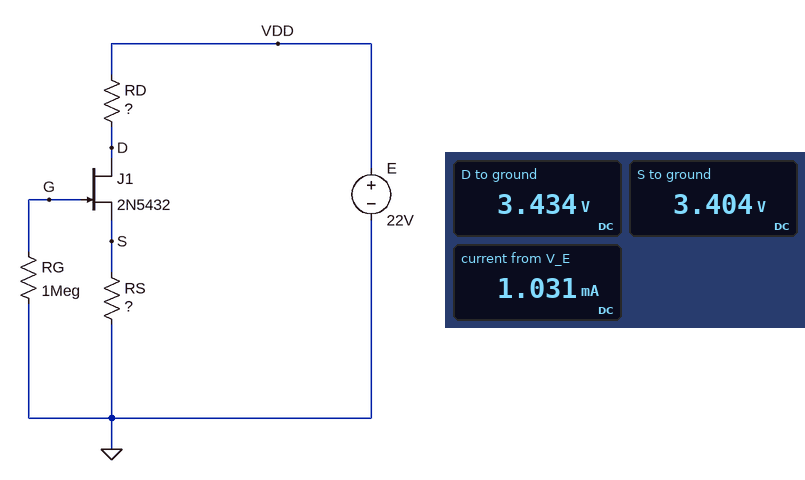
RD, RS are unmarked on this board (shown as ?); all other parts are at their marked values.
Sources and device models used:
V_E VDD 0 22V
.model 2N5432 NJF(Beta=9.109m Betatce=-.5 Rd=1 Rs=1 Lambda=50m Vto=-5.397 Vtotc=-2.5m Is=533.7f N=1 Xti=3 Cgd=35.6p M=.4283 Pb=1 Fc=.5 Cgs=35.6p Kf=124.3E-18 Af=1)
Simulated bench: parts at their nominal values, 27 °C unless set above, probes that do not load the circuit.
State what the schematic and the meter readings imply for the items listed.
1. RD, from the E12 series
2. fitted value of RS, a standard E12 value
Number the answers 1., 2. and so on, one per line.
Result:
1. 18 kΩ
2. 3.3 kΩ
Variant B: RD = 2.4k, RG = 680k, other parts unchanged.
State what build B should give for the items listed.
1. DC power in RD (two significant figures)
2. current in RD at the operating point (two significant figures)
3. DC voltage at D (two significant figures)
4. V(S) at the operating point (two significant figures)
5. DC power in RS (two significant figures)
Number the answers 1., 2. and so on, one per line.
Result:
1. 5.7 mW
2. 1.5 mA
3. 18 V
4. 5.1 V
5. 7.8 mW
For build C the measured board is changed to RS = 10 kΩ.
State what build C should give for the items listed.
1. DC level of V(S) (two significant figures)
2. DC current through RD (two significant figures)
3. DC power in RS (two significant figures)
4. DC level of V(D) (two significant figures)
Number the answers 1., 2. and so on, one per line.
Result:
1. 5.2 V
2. 520 µA
3. 2.7 mW
4. 13 V
